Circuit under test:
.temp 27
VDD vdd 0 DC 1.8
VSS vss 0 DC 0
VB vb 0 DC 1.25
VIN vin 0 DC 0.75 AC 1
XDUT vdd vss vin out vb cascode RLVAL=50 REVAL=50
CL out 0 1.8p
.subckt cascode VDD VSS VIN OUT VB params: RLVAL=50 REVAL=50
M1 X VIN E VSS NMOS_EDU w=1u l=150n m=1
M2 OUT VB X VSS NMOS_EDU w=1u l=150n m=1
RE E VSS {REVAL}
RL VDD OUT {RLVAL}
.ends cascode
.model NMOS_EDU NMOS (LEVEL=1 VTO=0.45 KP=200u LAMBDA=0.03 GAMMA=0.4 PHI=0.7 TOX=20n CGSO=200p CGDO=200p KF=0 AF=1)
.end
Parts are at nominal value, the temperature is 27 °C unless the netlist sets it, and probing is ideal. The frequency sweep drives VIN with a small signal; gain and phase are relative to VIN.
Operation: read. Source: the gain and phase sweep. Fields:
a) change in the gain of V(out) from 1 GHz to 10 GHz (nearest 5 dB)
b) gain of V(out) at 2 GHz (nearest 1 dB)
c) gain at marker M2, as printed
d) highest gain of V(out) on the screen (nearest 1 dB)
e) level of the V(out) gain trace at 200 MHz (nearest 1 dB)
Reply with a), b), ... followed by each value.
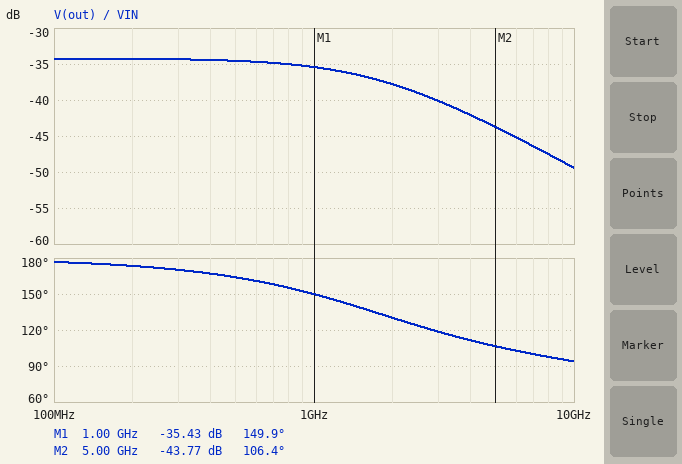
a) -15 dB
b) -38 dB
c) -43.77 dB
d) -34 dB
e) -34 dB
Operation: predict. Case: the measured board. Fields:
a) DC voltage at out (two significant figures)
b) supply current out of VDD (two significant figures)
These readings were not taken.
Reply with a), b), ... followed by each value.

a) 1.8 V
b) 59 µA
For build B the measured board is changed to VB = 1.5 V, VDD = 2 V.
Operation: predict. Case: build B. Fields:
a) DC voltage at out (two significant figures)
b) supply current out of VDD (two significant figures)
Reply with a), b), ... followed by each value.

a) 2.0 V
b) 60 µA
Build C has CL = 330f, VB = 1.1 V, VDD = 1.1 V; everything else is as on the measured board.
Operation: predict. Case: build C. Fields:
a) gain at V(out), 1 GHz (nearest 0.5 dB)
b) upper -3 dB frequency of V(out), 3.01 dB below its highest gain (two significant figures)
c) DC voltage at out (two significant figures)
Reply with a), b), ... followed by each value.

a) -34.5 dB
b) 9.6 GHz
c) 1.1 V
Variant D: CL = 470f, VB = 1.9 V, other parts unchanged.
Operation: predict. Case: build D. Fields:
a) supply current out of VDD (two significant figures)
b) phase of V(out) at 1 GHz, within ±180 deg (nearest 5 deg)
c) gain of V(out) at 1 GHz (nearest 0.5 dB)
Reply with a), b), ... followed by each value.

a) 60 µA
b) 170 deg
c) -34.0 dB
